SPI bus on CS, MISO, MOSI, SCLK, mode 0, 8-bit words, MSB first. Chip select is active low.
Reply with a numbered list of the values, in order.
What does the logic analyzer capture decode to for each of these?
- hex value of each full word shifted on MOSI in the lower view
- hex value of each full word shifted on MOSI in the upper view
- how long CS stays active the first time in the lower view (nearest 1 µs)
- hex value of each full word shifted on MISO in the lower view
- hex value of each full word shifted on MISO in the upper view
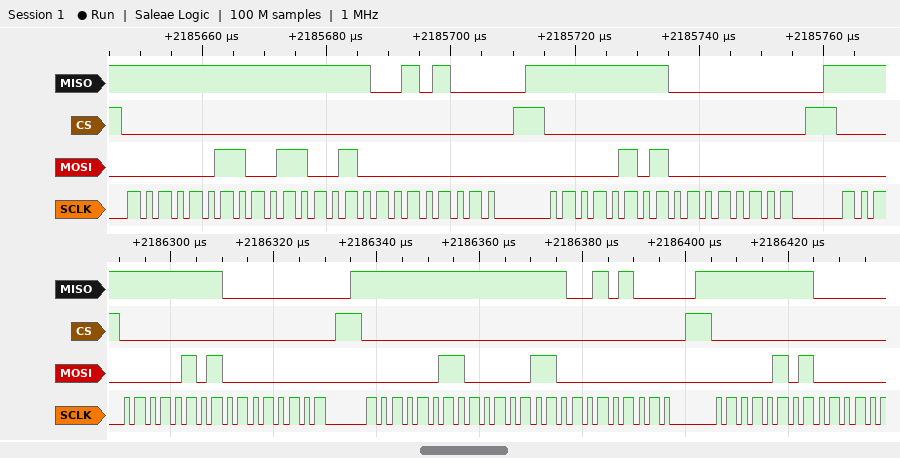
1. 05, 00, 03, 06, 00, 05
2. 03, 32, 00, 05, 00
3. 42 µs
4. FF, 00, FF, FF, 28, FF
5. FF, FF, 28, FF, 00
